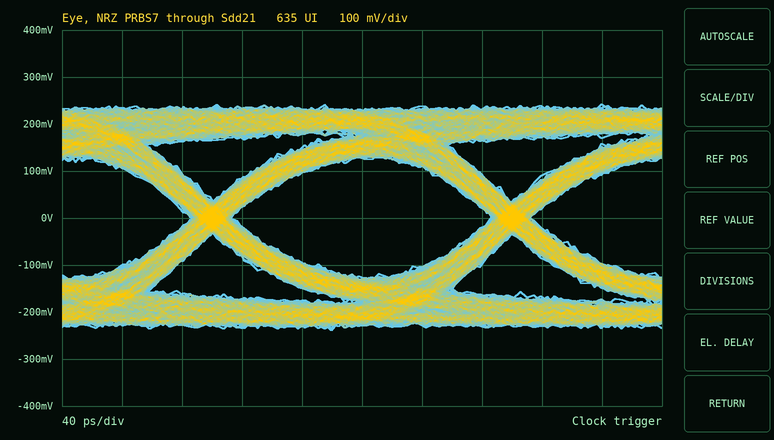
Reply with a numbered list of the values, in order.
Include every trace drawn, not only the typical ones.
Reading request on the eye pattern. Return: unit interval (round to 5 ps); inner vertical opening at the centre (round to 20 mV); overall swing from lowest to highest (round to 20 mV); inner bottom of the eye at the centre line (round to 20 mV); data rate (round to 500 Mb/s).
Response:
1. 200 ps
2. 260 mV
3. 480 mV
4. -120 mV
5. 5.0 Gb/s
